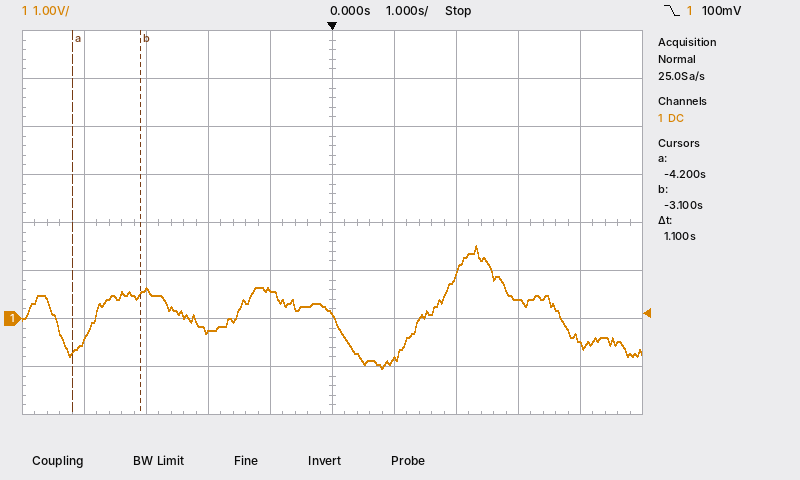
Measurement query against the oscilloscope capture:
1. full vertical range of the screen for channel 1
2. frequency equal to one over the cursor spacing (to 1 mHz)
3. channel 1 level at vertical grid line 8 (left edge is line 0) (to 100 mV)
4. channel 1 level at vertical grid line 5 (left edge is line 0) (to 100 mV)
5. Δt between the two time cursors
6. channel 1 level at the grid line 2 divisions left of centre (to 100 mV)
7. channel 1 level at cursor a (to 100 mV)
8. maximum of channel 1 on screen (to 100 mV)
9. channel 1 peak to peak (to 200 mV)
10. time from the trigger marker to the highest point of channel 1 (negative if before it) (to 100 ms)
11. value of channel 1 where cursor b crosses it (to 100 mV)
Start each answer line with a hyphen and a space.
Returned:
- 8 V
- 909 mHz
- 400 mV
- 100 mV
- 1.1 s
- -300 mV
- -700 mV
- 1.5 V
- 2.6 V
- +2.3 s
- 500 mV
